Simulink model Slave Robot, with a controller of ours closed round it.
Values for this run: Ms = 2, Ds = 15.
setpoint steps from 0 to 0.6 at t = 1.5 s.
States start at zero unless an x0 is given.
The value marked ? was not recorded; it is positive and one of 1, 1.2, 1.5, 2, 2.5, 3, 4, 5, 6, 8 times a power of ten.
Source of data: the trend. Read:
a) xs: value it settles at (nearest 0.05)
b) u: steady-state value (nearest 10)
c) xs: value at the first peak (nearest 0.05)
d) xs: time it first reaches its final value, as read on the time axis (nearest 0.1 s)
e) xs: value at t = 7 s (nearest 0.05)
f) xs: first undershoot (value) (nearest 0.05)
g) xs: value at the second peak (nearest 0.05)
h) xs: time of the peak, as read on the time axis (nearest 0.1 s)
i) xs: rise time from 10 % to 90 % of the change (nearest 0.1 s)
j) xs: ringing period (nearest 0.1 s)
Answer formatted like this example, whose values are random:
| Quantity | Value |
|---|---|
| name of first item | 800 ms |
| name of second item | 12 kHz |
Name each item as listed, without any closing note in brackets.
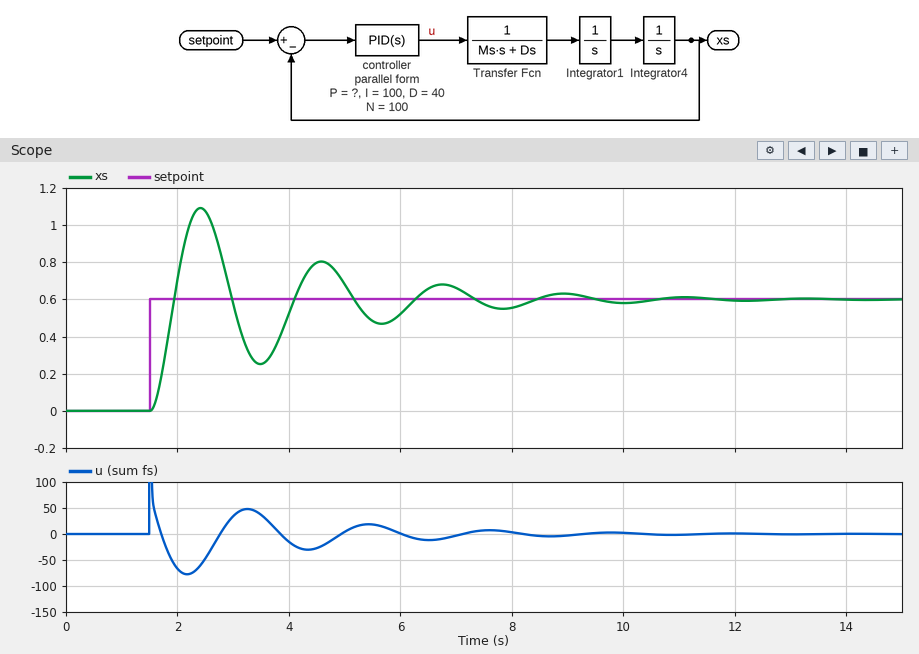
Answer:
| Quantity | Value |
|---|---|
| xs: value it settles at | 0.60 |
| u: steady-state value | 0 |
| xs: value at the first peak | 1.10 |
| xs: time it first reaches its final value, as read on the time axis | 1.9 s |
| xs: value at t = 7 s | 0.65 |
| xs: first undershoot (value) | 0.25 |
| xs: value at the second peak | 0.80 |
| xs: time of the peak, as read on the time axis | 2.4 s |
| xs: rise time from 10 % to 90 % of the change | 0.3 s |
| xs: ringing period | 2.2 s |
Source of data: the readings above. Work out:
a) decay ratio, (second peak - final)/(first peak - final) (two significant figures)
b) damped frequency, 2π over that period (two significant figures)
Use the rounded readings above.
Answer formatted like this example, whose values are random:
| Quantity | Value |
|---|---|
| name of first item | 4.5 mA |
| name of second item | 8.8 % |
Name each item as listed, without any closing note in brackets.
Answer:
| Quantity | Value |
|---|---|
| decay ratio, (second peak - final)/(first peak - final) | 0.40 |
| damped frequency, 2π over that period | 2.9 rad/s |
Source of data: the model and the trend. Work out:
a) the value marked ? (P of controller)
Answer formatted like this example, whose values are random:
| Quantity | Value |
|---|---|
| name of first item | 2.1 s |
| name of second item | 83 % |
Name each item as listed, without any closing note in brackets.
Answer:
| Quantity | Value |
|---|---|
| the value marked ? | 120 |
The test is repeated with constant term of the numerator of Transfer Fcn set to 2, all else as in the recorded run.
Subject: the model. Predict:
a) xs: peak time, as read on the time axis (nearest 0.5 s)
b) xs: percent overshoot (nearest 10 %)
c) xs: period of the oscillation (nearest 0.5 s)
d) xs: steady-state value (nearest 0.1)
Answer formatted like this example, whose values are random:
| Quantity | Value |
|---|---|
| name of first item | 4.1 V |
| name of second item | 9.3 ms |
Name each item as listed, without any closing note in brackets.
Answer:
| Quantity | Value |
|---|---|
| xs: peak time, as read on the time axis | 2.0 s |
| xs: percent overshoot | 70 % |
| xs: period of the oscillation | 1.5 s |
| xs: steady-state value | 0.6 |
